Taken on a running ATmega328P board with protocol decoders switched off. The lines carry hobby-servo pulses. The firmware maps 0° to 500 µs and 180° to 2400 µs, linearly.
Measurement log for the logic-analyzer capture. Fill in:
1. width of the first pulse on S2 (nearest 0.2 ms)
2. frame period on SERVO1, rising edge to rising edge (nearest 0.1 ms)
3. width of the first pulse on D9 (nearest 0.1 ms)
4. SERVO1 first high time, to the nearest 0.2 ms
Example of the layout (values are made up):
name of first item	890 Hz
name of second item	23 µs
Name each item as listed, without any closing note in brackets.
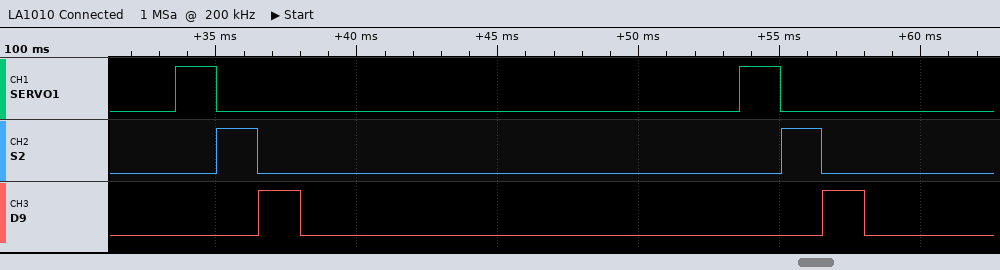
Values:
width of the first pulse on S2	1.4 ms
frame period on SERVO1, rising edge to rising edge	20.0 ms
width of the first pulse on D9	1.5 ms
SERVO1 first high time, to the nearest 0.2 ms	1.4 ms
